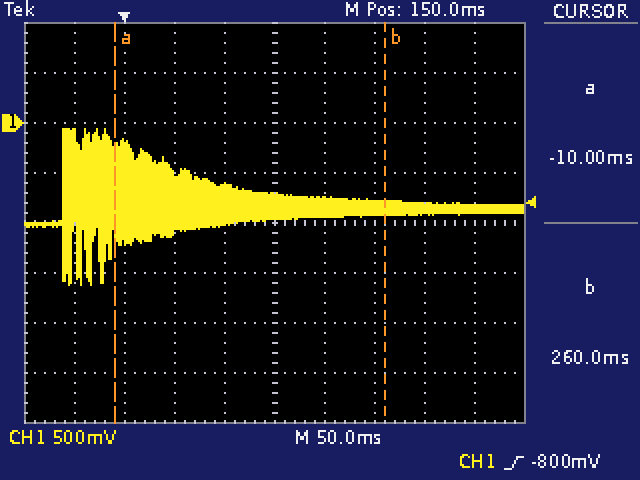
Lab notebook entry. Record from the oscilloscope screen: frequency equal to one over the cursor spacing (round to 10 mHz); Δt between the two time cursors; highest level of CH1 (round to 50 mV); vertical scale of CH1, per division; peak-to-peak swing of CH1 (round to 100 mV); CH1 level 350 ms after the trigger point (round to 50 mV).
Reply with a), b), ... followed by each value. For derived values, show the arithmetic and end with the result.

a) 1 / 270 ms ≈ 3.70 Hz
b) 260 ms − (-10 ms) = 270 ms
c) -50 mV
d) 500 mV
e) 1.60 V
f) -850 mV
